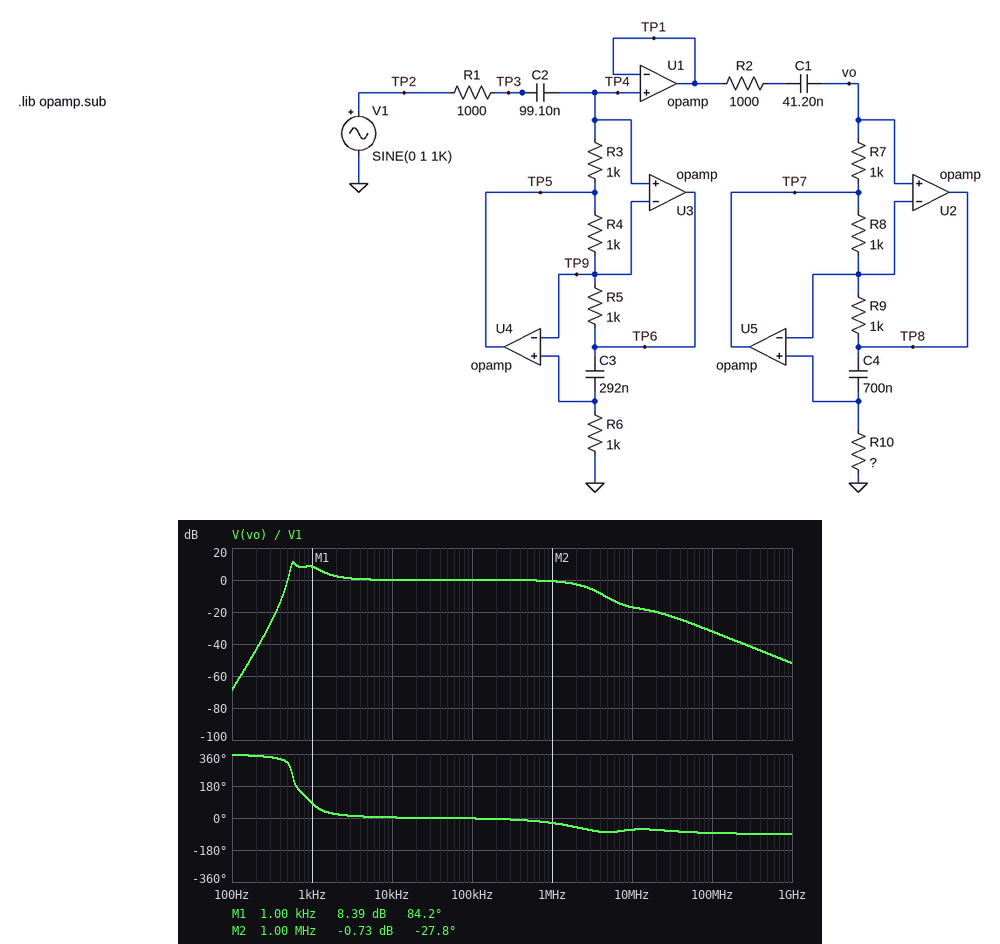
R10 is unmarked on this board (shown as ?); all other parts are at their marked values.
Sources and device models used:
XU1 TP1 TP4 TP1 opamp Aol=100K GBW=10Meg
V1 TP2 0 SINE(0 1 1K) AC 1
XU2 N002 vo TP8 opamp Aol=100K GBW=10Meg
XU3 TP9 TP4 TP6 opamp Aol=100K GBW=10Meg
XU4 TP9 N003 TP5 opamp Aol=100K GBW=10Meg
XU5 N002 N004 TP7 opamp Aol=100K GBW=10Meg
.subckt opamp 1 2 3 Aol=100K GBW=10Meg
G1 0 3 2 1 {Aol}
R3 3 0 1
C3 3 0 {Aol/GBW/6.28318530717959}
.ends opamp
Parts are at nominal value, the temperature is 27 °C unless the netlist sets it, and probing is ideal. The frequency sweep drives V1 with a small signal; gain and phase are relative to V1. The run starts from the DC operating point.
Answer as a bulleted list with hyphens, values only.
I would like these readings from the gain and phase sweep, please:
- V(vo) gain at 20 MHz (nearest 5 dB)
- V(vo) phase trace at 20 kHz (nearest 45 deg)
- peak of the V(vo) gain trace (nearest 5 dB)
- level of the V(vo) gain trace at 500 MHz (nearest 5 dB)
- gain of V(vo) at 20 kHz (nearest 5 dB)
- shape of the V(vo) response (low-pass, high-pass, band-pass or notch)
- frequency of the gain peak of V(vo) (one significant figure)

- -20 dB
- 0 deg
- 10 dB
- -45 dB
- 0 dB
- band-pass
- 600 Hz
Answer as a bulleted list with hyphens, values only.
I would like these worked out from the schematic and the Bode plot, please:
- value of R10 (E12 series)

- 2.7 kΩ
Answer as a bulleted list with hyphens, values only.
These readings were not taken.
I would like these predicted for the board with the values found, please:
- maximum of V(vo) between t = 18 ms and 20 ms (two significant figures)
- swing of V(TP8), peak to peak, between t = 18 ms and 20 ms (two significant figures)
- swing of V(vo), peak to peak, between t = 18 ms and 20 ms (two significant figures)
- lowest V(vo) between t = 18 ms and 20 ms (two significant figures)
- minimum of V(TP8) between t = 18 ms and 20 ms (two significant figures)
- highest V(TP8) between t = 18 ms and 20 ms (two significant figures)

- 2.6 V
- 5.3 V
- 5.3 V
- -2.6 V
- -2.6 V
- 2.6 V
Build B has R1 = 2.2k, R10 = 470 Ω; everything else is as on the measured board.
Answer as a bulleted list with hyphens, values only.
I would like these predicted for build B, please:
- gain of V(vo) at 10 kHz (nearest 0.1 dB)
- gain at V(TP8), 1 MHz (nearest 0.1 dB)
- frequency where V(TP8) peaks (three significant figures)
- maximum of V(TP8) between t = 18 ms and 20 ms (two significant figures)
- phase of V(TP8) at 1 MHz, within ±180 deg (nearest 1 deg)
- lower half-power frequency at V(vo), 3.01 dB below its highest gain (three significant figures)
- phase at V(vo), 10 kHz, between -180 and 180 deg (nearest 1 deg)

- 0.2 dB
- -1.3 dB
- 1.42 kHz
- 930 mV
- -40 deg
- 1.22 kHz
- 9 deg
